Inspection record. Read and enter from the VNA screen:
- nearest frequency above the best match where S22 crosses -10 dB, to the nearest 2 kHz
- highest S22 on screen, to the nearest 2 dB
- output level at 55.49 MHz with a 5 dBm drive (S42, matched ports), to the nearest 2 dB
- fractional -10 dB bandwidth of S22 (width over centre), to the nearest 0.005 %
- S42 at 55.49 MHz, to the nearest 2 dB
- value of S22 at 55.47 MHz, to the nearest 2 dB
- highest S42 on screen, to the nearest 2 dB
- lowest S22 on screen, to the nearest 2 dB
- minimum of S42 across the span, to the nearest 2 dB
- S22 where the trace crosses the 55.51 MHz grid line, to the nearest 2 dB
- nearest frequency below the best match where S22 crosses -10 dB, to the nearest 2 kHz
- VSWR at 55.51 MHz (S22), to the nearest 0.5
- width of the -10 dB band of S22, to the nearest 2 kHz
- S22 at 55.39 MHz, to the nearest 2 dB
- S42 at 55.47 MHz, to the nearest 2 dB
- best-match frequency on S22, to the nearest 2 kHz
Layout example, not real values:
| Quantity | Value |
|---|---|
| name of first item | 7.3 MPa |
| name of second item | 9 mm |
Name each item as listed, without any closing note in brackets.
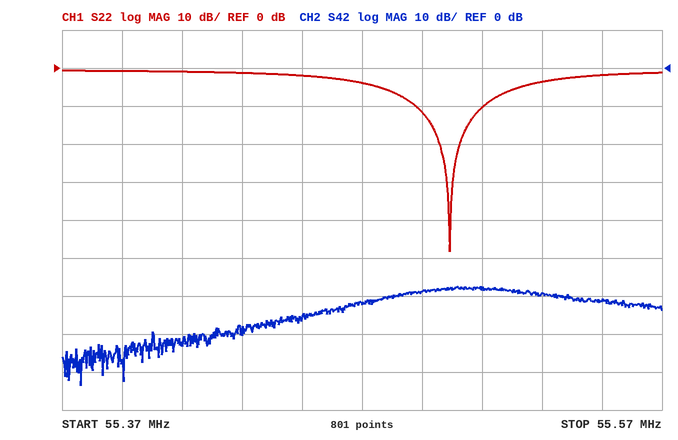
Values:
| Quantity | Value |
|---|---|
| nearest frequency above the best match where S22 crosses -10 dB, to the nearest 2 kHz | 55.510 MHz |
| highest S22 on screen, to the nearest 2 dB | 0 dB |
| output level at 55.49 MHz with a 5 dBm drive (S42, matched ports), to the nearest 2 dB | -54 dBm |
| fractional -10 dB bandwidth of S22 (width over centre), to the nearest 0.005 % | 0.040 % |
| S42 at 55.49 MHz, to the nearest 2 dB | -58 dB |
| value of S22 at 55.47 MHz, to the nearest 2 dB | -4 dB |
| highest S42 on screen, to the nearest 2 dB | -58 dB |
| lowest S22 on screen, to the nearest 2 dB | -48 dB |
| minimum of S42 across the span, to the nearest 2 dB | -84 dB |
| S22 where the trace crosses the 55.51 MHz grid line, to the nearest 2 dB | -10 dB |
| nearest frequency below the best match where S22 crosses -10 dB, to the nearest 2 kHz | 55.488 MHz |
| VSWR at 55.51 MHz (S22), to the nearest 0.5 | 2.0 |
| width of the -10 dB band of S22, to the nearest 2 kHz | 22 kHz |
| S22 at 55.39 MHz, to the nearest 2 dB | 0 dB |
| S42 at 55.47 MHz, to the nearest 2 dB | -62 dB |
| best-match frequency on S22, to the nearest 2 kHz | 55.500 MHz |
